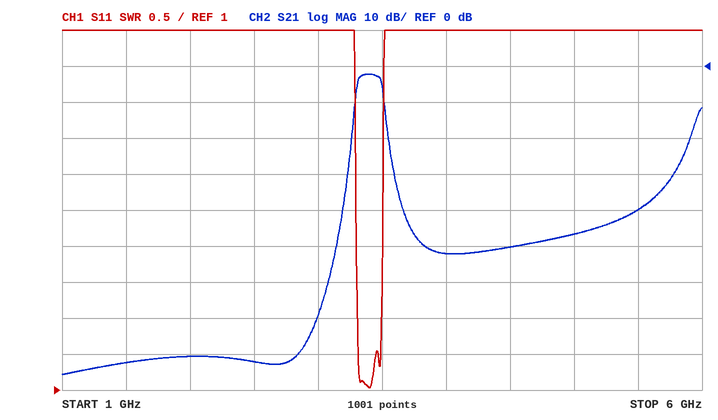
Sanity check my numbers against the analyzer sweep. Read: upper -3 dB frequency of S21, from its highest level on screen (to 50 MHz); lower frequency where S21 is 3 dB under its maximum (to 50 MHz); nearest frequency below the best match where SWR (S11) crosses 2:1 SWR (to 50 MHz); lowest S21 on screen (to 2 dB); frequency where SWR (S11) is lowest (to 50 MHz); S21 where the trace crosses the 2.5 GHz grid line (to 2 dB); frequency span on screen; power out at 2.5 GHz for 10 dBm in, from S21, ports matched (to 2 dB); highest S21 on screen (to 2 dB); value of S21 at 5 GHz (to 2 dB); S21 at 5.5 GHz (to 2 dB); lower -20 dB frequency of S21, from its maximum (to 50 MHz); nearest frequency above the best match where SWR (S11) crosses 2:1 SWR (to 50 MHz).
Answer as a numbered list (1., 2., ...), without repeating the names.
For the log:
1. 3.50 GHz
2. 3.30 GHz
3. 3.30 GHz
4. -86 dB
5. 3.40 GHz
6. -82 dB
7. 5 GHz
8. -72 dBm
9. -2 dB
10. -46 dB
11. -40 dB
12. 3.25 GHz
13. 3.50 GHz
